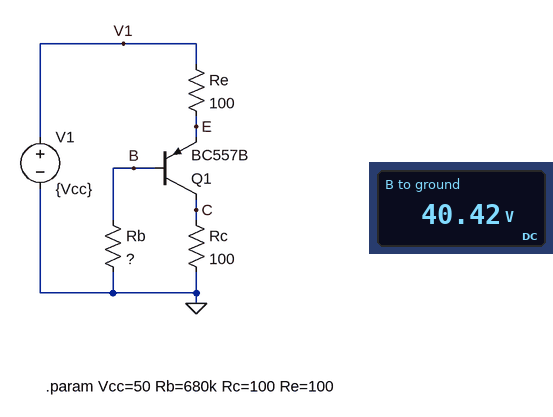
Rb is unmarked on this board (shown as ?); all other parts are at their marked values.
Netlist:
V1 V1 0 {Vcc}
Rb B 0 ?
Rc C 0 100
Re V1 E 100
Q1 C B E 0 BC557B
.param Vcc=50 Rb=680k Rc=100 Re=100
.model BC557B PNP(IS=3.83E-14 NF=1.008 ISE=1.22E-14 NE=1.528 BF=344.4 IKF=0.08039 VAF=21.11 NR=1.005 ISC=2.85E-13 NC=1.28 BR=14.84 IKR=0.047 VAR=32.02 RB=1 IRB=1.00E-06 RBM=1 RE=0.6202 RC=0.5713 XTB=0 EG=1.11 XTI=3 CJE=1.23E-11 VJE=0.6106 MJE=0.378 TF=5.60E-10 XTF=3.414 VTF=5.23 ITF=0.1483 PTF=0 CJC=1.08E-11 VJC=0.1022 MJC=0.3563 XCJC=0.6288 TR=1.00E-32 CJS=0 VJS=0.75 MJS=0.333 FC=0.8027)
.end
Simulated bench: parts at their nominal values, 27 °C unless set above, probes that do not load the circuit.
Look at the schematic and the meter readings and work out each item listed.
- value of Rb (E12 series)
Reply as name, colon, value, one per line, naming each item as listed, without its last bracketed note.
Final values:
value of Rb: 270 kΩ
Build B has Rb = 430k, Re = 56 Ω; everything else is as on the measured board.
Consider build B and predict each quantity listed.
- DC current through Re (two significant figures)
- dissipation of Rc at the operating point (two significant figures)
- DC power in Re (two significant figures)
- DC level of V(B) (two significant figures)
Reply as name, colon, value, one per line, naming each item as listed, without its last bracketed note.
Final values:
DC current through Re: 74 mA
dissipation of Rc at the operating point: 550 mW
DC power in Re: 310 mW
DC level of V(B): 45 V
